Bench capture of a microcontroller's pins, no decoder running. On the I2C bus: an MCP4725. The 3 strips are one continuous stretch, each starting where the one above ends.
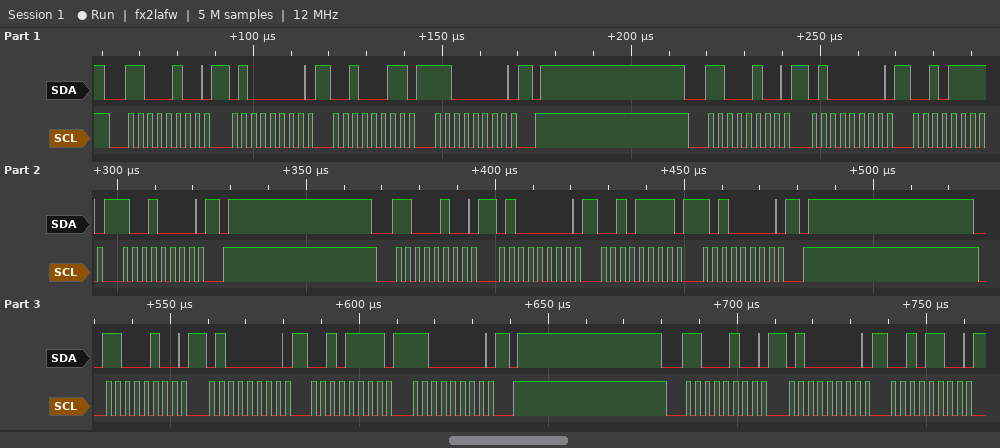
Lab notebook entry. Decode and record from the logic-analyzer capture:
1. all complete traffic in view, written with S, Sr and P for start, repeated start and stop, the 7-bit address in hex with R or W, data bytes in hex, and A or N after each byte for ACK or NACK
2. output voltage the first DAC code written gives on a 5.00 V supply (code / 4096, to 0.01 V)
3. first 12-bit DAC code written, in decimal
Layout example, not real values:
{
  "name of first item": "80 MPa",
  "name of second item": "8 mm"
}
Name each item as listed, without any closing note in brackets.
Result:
{
  "all complete traffic in view, written with S, Sr and P for start, repeated start and stop, the 7-bit address in hex with R or W, data bytes in hex, and A or N after each byte for ACK or NACK": "S 62W A 40 A 23 A C0 A P S 62W A 40 A 2F A 90 A P S 62W A 40 A 2F A A0 A P S 62W A 40 A 2F A C0 A P S 62W A 40 A 2C A",
  "output voltage the first DAC code written gives on a 5.00 V supply": "0.70 V",
  "first 12-bit DAC code written, in decimal": "572"
}
